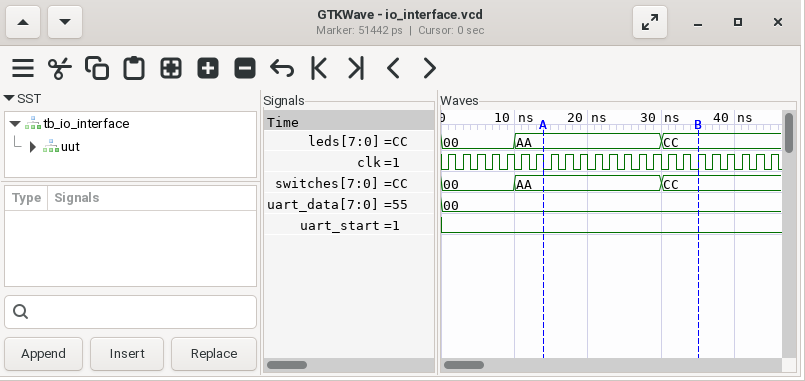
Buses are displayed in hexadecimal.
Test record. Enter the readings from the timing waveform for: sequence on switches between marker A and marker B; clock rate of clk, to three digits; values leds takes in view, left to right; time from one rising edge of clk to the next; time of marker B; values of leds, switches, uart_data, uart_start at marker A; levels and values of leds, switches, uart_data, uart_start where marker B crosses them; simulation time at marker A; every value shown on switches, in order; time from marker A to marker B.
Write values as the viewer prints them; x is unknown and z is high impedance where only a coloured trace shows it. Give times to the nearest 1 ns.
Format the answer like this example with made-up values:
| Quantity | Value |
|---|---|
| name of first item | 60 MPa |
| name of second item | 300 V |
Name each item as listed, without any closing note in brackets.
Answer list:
| Quantity | Value |
|---|---|
| sequence on switches between marker A and marker B | AA, CC |
| clock rate of clk, to three digits | 500 MHz |
| values leds takes in view, left to right | 00, AA, CC |
| time from one rising edge of clk to the next | 2 ns |
| time of marker B | 35 ns |
| values of leds, switches, uart_data, uart_start at marker A | leds=AA, switches=AA, uart_data=00, uart_start=0 |
| levels and values of leds, switches, uart_data, uart_start where marker B crosses them | leds=CC, switches=CC, uart_data=00, uart_start=0 |
| simulation time at marker A | 14 ns |
| every value shown on switches, in order | 00, AA, CC |
| time from marker A to marker B | 21 ns |
